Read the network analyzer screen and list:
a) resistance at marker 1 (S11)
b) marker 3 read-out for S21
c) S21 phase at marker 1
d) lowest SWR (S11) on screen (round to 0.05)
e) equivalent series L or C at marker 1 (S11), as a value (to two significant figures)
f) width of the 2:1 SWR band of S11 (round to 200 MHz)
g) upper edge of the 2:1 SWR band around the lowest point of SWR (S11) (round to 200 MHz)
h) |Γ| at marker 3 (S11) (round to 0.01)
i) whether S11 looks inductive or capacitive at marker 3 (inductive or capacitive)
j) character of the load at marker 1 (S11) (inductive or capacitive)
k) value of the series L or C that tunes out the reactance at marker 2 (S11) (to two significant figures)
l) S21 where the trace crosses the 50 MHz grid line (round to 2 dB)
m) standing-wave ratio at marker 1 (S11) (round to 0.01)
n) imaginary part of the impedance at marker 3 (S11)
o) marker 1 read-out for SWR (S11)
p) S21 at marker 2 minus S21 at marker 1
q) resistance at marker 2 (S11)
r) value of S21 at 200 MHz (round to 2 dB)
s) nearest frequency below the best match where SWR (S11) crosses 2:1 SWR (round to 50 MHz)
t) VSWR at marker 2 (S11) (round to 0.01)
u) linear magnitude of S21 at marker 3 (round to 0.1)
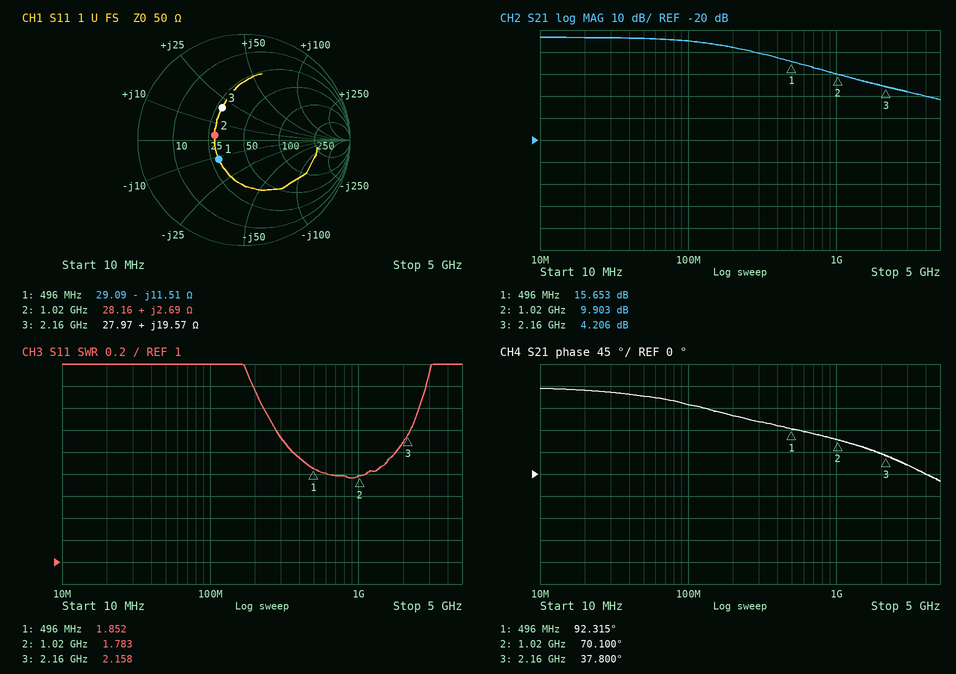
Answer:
29.09 Ω
4.206 dB
92.315°
1.75
28 pF
1.4 GHz
1.8 GHz
0.37
inductive
capacitive
58 pF
26 dB
1.85
+19.57 Ω
1.852
-5.750 dB
28.16 Ω
22 dB
350 MHz
1.78
1.6
